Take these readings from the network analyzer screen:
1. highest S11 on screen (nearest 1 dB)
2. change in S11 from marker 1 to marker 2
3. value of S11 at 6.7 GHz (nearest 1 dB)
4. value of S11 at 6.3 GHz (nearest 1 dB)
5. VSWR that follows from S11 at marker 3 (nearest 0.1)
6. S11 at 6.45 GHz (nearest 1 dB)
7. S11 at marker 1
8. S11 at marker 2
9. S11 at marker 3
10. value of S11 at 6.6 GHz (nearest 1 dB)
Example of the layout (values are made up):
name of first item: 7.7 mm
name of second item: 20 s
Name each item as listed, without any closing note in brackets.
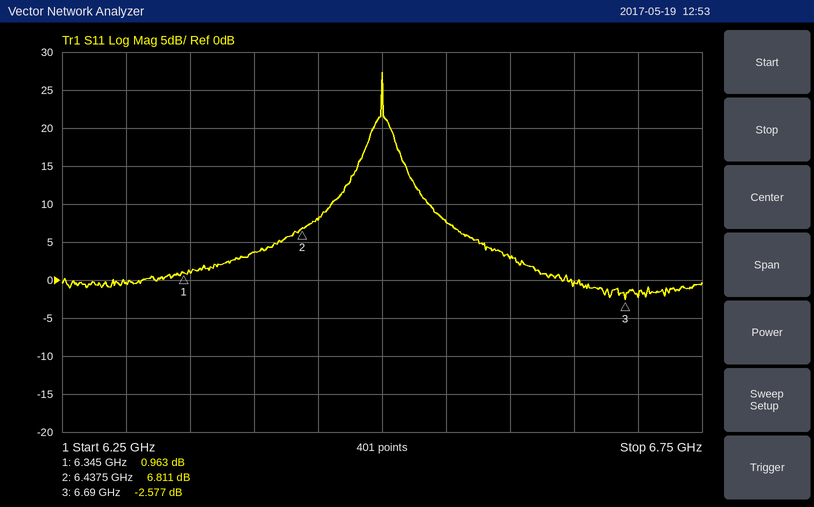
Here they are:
highest S11 on screen: 27 dB
change in S11 from marker 1 to marker 2: 5.848 dB
value of S11 at 6.7 GHz: -2 dB
value of S11 at 6.3 GHz: 0 dB
VSWR that follows from S11 at marker 3: 6.8
S11 at 6.45 GHz: 8 dB
S11 at marker 1: 0.963 dB
S11 at marker 2: 6.811 dB
S11 at marker 3: -2.577 dB
value of S11 at 6.6 GHz: 3 dB
